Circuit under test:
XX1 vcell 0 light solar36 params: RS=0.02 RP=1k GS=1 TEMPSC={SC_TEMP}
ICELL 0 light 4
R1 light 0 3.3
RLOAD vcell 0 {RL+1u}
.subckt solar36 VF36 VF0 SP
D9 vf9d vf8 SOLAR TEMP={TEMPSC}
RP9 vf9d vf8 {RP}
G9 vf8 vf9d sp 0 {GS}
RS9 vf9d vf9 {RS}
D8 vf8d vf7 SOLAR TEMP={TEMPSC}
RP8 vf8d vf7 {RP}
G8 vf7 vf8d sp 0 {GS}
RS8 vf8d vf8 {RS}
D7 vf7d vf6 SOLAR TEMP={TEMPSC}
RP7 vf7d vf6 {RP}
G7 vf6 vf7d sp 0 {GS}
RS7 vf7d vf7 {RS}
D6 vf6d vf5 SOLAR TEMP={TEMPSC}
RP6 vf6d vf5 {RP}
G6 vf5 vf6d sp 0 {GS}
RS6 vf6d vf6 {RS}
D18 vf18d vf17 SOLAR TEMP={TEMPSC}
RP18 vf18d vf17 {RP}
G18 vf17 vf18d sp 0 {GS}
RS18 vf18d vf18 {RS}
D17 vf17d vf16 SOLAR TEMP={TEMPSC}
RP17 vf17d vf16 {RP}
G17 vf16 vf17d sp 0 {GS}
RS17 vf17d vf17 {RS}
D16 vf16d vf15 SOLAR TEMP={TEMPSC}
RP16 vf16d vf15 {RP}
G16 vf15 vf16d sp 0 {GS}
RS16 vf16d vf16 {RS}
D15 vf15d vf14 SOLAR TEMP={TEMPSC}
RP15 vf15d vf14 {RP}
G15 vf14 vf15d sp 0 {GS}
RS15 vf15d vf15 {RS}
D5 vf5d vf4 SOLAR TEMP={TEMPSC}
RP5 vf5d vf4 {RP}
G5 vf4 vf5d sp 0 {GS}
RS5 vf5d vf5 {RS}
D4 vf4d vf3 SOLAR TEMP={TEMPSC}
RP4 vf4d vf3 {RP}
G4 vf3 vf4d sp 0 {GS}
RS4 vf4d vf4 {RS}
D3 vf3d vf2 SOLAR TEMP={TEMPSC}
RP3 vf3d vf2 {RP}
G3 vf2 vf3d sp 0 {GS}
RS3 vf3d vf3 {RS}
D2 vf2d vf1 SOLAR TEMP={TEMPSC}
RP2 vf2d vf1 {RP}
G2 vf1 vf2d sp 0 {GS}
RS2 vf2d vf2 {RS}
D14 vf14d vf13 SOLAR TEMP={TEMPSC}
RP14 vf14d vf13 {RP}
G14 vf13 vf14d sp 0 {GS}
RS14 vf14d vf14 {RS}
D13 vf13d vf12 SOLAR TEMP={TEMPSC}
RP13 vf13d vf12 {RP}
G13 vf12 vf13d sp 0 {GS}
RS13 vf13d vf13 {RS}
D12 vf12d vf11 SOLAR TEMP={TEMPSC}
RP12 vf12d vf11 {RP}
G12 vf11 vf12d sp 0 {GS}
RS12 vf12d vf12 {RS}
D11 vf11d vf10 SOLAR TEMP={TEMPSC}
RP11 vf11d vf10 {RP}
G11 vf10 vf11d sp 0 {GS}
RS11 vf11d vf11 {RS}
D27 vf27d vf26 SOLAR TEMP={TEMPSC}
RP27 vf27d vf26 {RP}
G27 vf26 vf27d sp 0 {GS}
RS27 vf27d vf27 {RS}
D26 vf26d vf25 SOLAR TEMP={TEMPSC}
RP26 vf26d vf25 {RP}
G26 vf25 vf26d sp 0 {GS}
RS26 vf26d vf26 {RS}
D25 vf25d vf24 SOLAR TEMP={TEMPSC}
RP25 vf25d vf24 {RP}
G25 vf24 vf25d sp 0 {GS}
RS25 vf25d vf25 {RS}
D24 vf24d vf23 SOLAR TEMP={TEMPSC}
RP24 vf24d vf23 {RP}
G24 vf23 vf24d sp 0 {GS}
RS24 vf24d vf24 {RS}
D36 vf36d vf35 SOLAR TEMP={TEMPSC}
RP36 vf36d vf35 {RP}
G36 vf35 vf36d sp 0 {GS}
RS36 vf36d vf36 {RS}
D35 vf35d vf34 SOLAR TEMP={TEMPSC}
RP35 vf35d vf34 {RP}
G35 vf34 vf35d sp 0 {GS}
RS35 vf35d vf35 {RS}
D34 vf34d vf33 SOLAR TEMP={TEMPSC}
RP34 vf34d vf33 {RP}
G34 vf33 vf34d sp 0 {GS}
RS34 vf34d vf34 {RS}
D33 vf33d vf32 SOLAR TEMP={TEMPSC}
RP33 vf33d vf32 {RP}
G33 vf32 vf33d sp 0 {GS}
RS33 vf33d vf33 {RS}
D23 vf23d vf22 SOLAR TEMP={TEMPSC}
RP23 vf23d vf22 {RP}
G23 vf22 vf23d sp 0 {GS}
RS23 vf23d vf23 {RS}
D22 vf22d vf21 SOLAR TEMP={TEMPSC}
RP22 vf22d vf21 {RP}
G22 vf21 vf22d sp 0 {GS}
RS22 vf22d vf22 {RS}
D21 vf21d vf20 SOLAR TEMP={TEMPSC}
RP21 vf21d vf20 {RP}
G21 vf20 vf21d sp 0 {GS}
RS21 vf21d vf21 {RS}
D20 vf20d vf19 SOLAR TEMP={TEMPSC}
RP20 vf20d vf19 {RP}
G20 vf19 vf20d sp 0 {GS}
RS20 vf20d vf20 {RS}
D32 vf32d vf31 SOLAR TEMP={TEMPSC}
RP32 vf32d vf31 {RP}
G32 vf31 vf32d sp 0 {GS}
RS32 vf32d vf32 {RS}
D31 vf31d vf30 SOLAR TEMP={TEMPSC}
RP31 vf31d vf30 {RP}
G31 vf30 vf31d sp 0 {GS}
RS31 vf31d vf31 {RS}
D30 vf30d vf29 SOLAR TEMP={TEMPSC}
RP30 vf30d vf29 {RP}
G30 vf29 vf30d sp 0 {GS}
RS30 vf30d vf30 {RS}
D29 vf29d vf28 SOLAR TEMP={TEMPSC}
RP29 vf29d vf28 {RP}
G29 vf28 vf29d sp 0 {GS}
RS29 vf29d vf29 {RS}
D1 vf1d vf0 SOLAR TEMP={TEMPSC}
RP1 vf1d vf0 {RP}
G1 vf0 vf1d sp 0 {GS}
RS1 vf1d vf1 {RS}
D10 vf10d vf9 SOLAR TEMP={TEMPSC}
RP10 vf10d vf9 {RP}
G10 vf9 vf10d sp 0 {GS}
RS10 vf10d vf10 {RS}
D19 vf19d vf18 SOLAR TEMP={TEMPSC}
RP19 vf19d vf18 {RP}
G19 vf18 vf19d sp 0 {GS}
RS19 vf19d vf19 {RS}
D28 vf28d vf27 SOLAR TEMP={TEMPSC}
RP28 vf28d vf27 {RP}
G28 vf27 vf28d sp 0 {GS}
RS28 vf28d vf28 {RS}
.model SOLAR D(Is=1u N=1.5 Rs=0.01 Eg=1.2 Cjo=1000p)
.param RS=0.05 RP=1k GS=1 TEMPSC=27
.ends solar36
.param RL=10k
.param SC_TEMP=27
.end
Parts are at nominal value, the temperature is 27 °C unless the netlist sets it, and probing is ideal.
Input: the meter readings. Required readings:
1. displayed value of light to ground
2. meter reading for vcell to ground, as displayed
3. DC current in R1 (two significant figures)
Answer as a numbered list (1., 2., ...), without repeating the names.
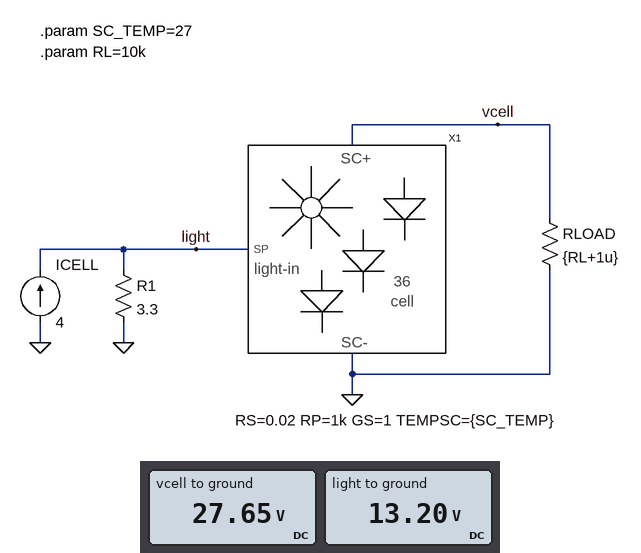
1. 13.20 V
2. 27.65 V
3. 4.0 A
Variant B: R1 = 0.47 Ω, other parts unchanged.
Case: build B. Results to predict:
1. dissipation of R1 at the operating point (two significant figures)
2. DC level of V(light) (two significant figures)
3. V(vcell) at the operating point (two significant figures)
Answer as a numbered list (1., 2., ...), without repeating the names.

1. 7.5 W
2. 1.9 V
3. 21 V
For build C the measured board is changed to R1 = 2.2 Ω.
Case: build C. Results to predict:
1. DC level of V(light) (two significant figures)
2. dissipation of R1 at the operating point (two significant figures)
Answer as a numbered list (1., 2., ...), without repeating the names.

1. 8.8 V
2. 35 W
